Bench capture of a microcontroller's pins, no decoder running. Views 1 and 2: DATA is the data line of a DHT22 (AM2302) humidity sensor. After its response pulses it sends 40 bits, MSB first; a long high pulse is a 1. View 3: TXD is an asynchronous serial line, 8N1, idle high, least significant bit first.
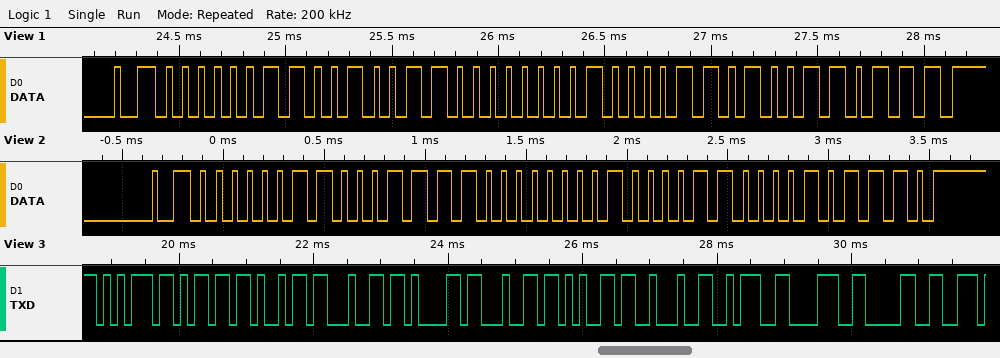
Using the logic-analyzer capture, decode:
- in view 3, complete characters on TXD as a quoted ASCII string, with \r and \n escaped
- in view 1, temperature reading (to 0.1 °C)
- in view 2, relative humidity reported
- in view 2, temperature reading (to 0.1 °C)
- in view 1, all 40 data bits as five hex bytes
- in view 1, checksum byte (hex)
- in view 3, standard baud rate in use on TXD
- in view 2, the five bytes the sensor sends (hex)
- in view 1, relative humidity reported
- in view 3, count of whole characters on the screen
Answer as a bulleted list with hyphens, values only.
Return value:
- "umidade\":80"
- 26.9 °C
- 79.8 %
- 26.8 °C
- 03 26 01 0D 37
- 0x37
- 9600 baud
- 03 1E 01 0C 2E
- 80.6 %
- 11
